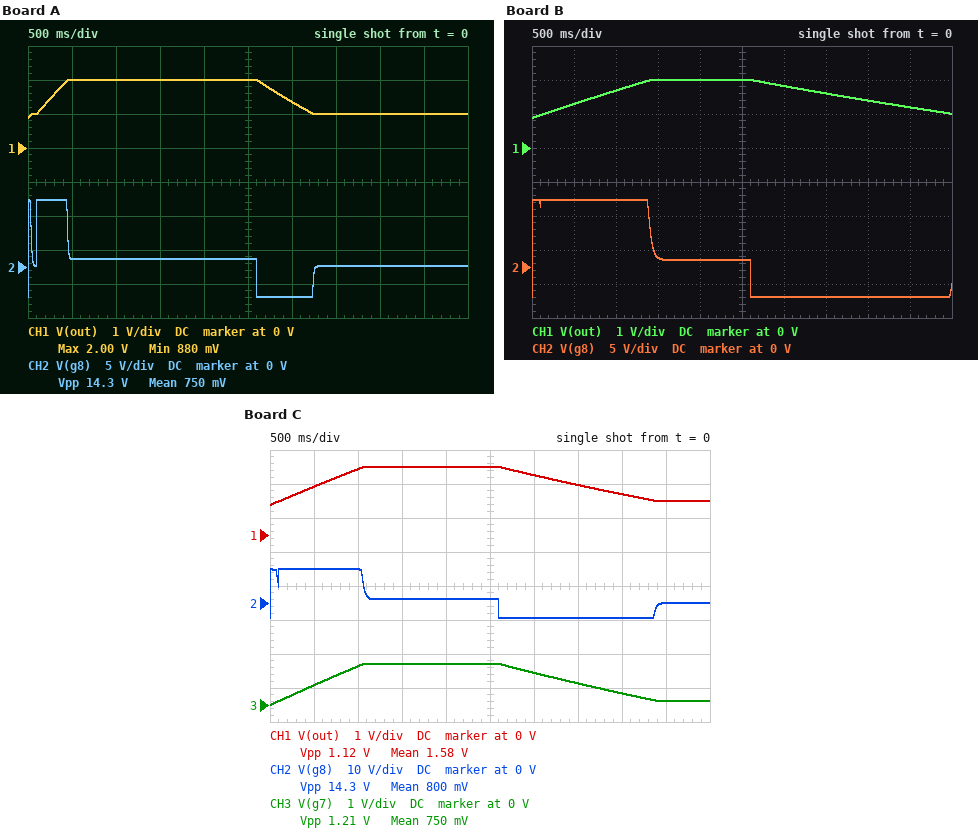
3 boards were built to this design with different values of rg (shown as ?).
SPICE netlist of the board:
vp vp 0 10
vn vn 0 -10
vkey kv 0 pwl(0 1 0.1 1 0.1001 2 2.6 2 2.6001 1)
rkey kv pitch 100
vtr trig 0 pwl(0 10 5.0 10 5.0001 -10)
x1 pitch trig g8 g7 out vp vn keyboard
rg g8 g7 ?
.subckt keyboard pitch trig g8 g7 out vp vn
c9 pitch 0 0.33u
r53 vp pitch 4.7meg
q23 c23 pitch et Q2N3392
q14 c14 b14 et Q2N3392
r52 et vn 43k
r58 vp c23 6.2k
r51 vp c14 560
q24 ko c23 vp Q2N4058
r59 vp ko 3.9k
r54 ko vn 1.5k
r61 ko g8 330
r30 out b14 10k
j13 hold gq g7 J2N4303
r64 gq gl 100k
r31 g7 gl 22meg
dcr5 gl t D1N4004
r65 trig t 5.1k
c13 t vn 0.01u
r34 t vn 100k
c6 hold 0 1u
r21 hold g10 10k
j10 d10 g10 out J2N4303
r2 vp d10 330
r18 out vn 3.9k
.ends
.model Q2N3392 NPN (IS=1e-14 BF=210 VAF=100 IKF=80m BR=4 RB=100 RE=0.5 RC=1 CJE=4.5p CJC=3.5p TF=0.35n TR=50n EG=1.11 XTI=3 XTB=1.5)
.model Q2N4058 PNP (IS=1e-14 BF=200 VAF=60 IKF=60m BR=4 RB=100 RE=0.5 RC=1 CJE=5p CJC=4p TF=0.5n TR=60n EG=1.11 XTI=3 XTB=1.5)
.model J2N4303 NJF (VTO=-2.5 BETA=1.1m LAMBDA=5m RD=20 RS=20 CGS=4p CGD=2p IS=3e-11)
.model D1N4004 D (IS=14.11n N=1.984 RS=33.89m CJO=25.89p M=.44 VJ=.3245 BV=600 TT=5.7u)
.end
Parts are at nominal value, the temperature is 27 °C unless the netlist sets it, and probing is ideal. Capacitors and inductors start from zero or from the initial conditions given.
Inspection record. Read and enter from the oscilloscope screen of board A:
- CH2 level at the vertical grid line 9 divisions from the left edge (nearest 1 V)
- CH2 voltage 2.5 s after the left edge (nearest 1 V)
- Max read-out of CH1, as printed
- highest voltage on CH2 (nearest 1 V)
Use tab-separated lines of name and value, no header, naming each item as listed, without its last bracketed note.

CH2 level at the vertical grid line 9 divisions from the left edge	0 V
CH2 voltage 2.5 s after the left edge	1 V
Max read-out of CH1, as printed	2.00 V
highest voltage on CH2	10 V
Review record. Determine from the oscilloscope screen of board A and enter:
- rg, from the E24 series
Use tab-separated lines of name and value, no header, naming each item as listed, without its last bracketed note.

rg, from the E24 series	3 MΩ
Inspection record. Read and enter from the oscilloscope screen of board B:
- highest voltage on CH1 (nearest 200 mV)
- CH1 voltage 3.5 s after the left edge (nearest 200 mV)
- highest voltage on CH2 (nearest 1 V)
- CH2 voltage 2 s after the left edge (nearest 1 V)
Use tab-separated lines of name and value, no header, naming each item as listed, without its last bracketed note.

highest voltage on CH1	2.0 V
CH1 voltage 3.5 s after the left edge	1.6 V
highest voltage on CH2	10 V
CH2 voltage 2 s after the left edge	1 V
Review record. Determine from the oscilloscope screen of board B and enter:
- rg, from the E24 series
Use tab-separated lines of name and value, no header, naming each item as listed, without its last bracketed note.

rg, from the E24 series	11 MΩ
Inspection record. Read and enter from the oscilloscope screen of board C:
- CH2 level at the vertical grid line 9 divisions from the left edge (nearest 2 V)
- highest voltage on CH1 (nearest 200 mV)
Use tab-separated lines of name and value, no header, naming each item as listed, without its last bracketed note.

CH2 level at the vertical grid line 9 divisions from the left edge	0 V
highest voltage on CH1	2.0 V
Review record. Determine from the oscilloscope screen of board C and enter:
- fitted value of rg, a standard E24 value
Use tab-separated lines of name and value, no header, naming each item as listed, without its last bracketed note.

fitted value of rg, a standard E24 value	8.2 MΩ
